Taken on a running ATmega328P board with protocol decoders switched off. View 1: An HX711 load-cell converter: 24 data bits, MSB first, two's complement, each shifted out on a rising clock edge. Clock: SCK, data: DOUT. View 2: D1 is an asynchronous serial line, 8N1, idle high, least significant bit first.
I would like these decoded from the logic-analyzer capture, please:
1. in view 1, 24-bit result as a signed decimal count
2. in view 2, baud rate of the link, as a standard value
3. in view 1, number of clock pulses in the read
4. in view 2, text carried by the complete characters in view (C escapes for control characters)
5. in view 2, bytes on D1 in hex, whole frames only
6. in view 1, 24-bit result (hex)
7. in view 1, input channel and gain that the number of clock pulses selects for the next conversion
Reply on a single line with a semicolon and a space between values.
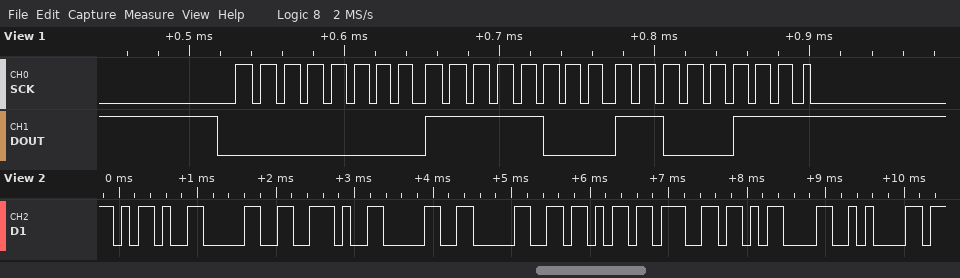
63687; 9600 baud; 25; "-0.00kg\r\n"; 0x2D 0x30 0x2E 0x30 0x30 0x6B 0x67 0x0D 0x0A; 0x00F8C7; channel A, gain 128
